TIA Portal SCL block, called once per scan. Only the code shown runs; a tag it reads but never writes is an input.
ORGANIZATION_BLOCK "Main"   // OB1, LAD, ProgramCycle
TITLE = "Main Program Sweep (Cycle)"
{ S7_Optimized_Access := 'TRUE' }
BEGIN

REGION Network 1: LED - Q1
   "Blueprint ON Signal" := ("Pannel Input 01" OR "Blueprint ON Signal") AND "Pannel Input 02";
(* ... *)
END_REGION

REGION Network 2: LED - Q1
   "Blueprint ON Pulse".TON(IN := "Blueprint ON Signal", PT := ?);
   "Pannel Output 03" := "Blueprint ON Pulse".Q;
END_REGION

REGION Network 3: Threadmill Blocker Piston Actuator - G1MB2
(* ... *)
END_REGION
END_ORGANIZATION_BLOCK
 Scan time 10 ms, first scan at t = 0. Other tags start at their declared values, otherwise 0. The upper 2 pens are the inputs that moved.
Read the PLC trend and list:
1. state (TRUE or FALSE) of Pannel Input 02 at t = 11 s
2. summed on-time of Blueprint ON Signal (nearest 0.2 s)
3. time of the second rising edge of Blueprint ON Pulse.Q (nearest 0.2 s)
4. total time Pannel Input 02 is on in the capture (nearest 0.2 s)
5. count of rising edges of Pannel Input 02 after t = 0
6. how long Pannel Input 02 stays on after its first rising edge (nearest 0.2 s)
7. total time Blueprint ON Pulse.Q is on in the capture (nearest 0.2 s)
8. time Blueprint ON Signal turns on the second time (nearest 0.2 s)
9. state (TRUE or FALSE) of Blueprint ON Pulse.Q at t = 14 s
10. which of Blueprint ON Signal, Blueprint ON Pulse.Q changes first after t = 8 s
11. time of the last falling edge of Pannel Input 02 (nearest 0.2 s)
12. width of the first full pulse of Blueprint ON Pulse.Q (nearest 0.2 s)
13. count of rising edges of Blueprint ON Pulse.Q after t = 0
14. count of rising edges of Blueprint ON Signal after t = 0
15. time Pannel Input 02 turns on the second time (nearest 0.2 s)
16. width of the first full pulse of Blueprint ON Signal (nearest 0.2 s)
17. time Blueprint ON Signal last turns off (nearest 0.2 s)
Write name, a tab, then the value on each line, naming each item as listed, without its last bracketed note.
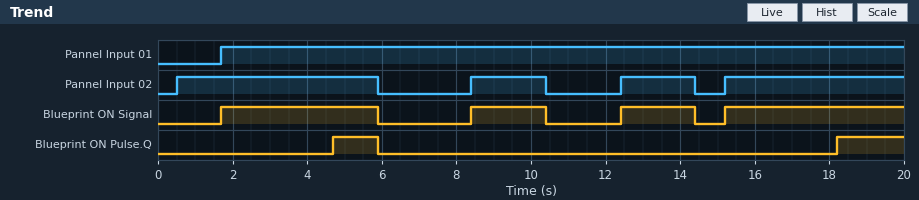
state (TRUE or FALSE) of Pannel Input 02 at t = 11 s	FALSE
summed on-time of Blueprint ON Signal	13.0 s
time of the second rising edge of Blueprint ON Pulse.Q	18.2 s
total time Pannel Input 02 is on in the capture	14.2 s
count of rising edges of Pannel Input 02 after t = 0	4
how long Pannel Input 02 stays on after its first rising edge	5.4 s
total time Blueprint ON Pulse.Q is on in the capture	3.0 s
time Blueprint ON Signal turns on the second time	8.4 s
state (TRUE or FALSE) of Blueprint ON Pulse.Q at t = 14 s	FALSE
which of Blueprint ON Signal, Blueprint ON Pulse.Q changes first after t = 8 s	Blueprint ON Signal
time of the last falling edge of Pannel Input 02	14.4 s
width of the first full pulse of Blueprint ON Pulse.Q	1.2 s
count of rising edges of Blueprint ON Pulse.Q after t = 0	2
count of rising edges of Blueprint ON Signal after t = 0	4
time Pannel Input 02 turns on the second time	8.4 s
width of the first full pulse of Blueprint ON Signal	4.2 s
time Blueprint ON Signal last turns off	14.4 s
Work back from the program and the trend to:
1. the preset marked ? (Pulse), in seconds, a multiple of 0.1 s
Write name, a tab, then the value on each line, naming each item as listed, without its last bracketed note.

the preset marked ? (Pulse), in seconds, a multiple of 0.1 s	3.0 s
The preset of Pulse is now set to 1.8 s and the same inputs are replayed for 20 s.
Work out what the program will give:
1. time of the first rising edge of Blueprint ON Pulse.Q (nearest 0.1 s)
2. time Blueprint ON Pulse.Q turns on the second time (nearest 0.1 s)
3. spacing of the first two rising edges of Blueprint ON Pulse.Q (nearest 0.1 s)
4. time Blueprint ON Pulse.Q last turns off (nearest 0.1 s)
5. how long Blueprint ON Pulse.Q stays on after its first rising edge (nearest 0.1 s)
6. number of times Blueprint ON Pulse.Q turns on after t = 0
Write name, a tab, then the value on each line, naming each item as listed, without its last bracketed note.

time of the first rising edge of Blueprint ON Pulse.Q	3.5 s
time Blueprint ON Pulse.Q turns on the second time	10.2 s
spacing of the first two rising edges of Blueprint ON Pulse.Q	6.7 s
time Blueprint ON Pulse.Q last turns off	14.4 s
how long Blueprint ON Pulse.Q stays on after its first rising edge	2.4 s
number of times Blueprint ON Pulse.Q turns on after t = 0	4
